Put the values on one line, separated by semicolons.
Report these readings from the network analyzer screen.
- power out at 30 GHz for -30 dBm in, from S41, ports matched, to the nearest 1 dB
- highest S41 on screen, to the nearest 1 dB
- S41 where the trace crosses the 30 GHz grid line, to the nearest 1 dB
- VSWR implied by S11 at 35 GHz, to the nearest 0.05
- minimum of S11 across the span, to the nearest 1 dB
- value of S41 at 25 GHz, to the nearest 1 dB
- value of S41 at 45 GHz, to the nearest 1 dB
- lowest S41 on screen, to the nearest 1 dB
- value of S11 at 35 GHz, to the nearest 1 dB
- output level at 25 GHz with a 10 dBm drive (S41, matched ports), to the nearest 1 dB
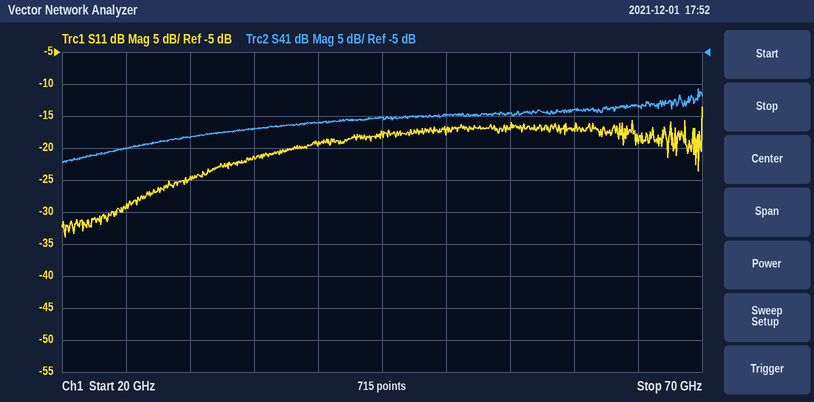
-48 dBm; -11 dB; -18 dB; 1.20; -34 dB; -20 dB; -15 dB; -22 dB; -21 dB; -10 dBm
